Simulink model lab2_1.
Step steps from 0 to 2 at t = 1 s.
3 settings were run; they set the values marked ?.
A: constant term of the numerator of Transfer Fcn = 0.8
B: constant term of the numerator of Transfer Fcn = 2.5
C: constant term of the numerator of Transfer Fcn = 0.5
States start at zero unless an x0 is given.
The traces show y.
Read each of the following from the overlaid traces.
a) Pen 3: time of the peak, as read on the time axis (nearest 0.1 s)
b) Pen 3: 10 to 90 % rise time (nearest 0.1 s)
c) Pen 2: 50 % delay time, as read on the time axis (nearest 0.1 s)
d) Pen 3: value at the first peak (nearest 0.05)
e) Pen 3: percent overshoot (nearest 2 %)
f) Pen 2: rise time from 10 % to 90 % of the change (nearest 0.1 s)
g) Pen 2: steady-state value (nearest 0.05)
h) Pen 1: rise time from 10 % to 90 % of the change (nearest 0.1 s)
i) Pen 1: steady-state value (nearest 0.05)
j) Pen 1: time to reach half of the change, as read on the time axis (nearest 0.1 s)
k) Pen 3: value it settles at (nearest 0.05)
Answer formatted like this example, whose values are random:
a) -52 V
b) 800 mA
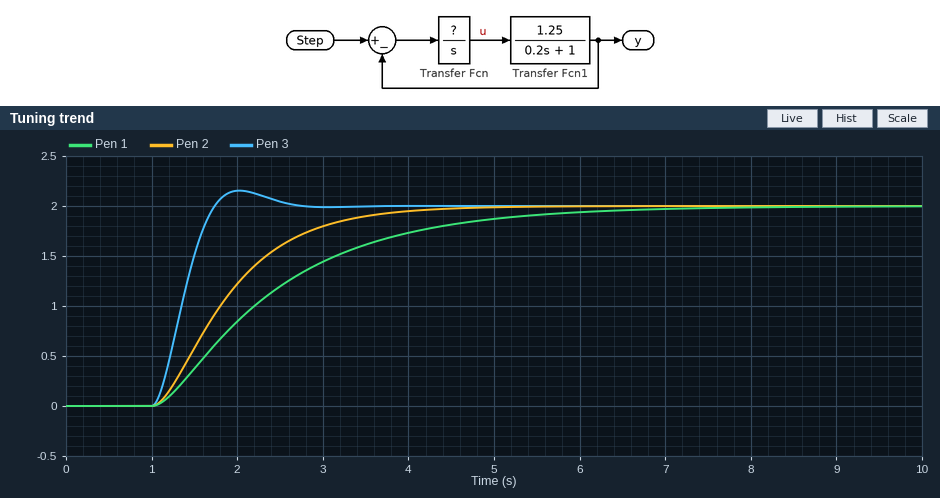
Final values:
a) 2.0 s
b) 0.5 s
c) 1.8 s
d) 2.15
e) 8 %
f) 1.8 s
g) 2.00
h) 3.1 s
i) 2.00
j) 2.2 s
k) 2.00
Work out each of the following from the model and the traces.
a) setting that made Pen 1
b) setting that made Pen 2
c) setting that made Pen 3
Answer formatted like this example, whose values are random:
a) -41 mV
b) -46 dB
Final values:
a) C
b) A
c) B
